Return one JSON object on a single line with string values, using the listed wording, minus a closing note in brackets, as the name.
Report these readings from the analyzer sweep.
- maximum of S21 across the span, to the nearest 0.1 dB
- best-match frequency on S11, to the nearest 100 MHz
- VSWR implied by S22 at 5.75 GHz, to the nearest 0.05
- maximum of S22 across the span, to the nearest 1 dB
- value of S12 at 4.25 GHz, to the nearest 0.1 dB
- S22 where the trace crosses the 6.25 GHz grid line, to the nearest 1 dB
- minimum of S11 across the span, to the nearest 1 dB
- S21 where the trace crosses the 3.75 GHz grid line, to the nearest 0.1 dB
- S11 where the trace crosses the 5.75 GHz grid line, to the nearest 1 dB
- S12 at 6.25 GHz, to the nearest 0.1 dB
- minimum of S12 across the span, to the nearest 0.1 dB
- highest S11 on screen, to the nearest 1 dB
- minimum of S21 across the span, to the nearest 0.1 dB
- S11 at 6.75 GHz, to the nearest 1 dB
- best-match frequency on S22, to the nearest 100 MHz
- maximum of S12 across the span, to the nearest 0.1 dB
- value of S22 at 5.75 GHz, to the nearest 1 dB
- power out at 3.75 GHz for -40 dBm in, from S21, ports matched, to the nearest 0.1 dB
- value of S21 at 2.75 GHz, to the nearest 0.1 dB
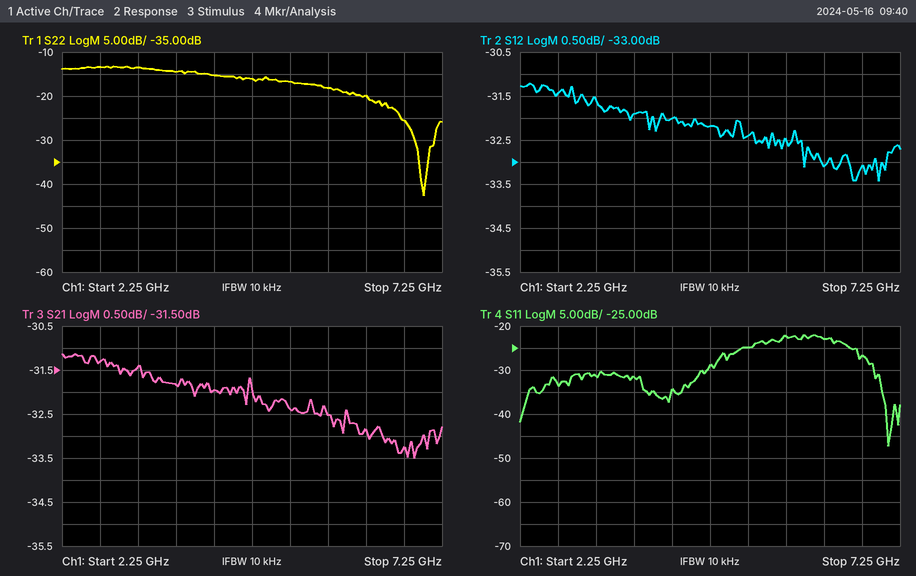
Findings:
{"maximum of S21 across the span, to the nearest 0.1 dB": "-31.1 dB", "best-match frequency on S11, to the nearest 100 MHz": "7.1 GHz", "VSWR implied by S22 at 5.75 GHz, to the nearest 0.05": "1.30", "maximum of S22 across the span, to the nearest 1 dB": "-13 dB", "value of S12 at 4.25 GHz, to the nearest 0.1 dB": "-32.0 dB", "S22 where the trace crosses the 6.25 GHz grid line, to the nearest 1 dB": "-20 dB", "minimum of S11 across the span, to the nearest 1 dB": "-47 dB", "S21 where the trace crosses the 3.75 GHz grid line, to the nearest 0.1 dB": "-31.8 dB", "S11 where the trace crosses the 5.75 GHz grid line, to the nearest 1 dB": "-22 dB", "S12 at 6.25 GHz, to the nearest 0.1 dB": "-33.1 dB", "minimum of S12 across the span, to the nearest 0.1 dB": "-33.4 dB", "highest S11 on screen, to the nearest 1 dB": "-22 dB", "minimum of S21 across the span, to the nearest 0.1 dB": "-33.5 dB", "S11 at 6.75 GHz, to the nearest 1 dB": "-27 dB", "best-match frequency on S22, to the nearest 100 MHz": "7.0 GHz", "maximum of S12 across the span, to the nearest 0.1 dB": "-31.2 dB", "value of S22 at 5.75 GHz, to the nearest 1 dB": "-18 dB", "power out at 3.75 GHz for -40 dBm in, from S21, ports matched, to the nearest 0.1 dB": "-71.8 dBm", "value of S21 at 2.75 GHz, to the nearest 0.1 dB": "-31.3 dB"}
